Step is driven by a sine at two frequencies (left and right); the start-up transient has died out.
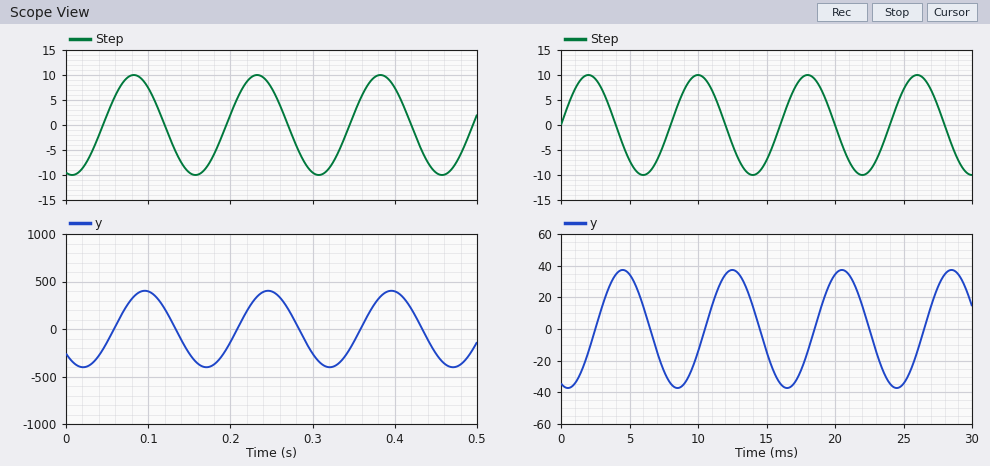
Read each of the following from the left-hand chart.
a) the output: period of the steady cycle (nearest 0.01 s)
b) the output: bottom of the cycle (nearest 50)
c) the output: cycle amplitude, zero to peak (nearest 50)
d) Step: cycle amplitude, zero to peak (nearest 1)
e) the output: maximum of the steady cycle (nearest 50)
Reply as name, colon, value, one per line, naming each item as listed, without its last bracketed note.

the output: period of the steady cycle: 0.15 s
the output: bottom of the cycle: -400
the output: cycle amplitude, zero to peak: 400
Step: cycle amplitude, zero to peak: 10
the output: maximum of the steady cycle: 400
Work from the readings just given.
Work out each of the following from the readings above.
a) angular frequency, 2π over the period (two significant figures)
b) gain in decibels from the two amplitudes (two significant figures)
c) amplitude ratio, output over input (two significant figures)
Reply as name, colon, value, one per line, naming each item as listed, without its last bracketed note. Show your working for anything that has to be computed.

angular frequency, 2π over the period: 2π / 0.15 = 42 rad/s
gain in decibels from the two amplitudes: 20 log10(400 / 10) = 32 dB
amplitude ratio, output over input: 400 / 10 = 40
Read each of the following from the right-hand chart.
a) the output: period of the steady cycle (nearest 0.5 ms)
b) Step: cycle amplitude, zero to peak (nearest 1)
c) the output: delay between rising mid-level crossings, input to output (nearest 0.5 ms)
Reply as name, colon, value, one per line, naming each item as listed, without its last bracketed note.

the output: period of the steady cycle: 8.0 ms
Step: cycle amplitude, zero to peak: 10
the output: delay between rising mid-level crossings, input to output: 2.5 ms
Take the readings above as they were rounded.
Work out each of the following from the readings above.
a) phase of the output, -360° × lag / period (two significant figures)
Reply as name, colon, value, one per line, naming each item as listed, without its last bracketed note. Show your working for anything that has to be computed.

phase of the output, -360° × lag / period: -360 × 2.5 / 8 = -110°
